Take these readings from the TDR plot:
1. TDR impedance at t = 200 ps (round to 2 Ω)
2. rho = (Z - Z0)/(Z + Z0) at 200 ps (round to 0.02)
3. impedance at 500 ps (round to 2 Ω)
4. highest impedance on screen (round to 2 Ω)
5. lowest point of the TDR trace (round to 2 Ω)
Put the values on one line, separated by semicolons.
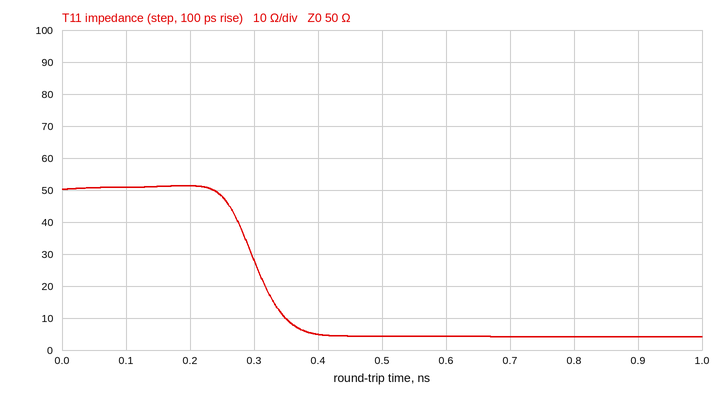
52 Ω; +0.02; 4 Ω; 52 Ω; 4 Ω
